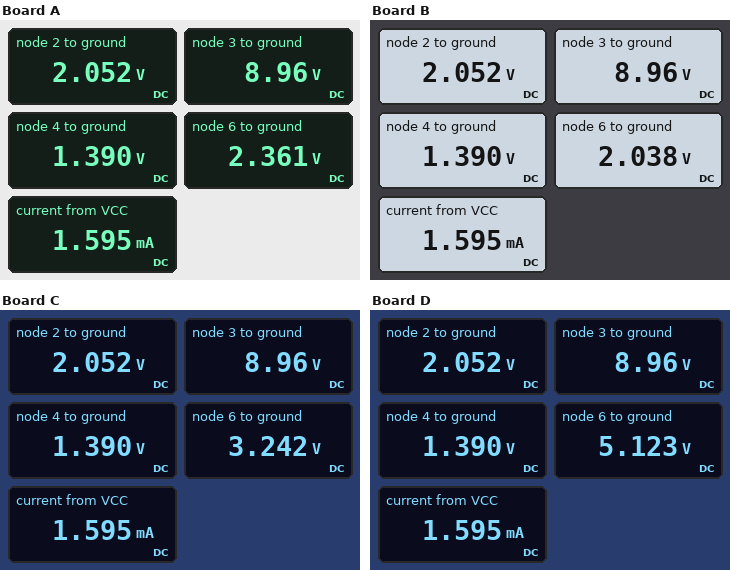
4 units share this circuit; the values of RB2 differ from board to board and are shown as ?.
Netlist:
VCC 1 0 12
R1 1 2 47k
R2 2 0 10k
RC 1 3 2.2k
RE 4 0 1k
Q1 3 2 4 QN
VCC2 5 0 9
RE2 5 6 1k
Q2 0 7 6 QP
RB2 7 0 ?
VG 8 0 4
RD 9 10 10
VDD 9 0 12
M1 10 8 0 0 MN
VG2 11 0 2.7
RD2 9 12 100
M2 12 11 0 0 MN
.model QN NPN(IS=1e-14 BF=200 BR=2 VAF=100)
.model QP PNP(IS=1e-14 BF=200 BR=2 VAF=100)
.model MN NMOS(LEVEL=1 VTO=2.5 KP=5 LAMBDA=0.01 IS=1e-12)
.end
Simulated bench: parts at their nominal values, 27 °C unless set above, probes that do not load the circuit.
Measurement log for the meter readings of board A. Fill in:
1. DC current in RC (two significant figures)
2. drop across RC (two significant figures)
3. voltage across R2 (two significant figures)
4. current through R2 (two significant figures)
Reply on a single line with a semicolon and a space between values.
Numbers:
1.4 mA; 3.0 V; 2.1 V; 210 µA
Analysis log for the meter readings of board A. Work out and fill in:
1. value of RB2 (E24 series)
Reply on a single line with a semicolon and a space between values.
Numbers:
51 kΩ
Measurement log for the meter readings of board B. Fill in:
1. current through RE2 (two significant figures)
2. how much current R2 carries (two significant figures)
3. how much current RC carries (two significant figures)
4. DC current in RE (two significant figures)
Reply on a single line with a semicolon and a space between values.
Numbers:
7.0 mA; 210 µA; 1.4 mA; 1.4 mA
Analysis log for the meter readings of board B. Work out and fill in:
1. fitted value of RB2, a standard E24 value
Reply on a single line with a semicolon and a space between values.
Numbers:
39 kΩ
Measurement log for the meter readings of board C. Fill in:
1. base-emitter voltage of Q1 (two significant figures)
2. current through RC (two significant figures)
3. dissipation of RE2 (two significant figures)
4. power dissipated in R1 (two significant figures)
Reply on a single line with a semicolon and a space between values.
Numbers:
660 mV; 1.4 mA; 33 mW; 2.1 mW
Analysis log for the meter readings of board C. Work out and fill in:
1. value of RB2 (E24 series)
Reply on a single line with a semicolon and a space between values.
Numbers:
91 kΩ
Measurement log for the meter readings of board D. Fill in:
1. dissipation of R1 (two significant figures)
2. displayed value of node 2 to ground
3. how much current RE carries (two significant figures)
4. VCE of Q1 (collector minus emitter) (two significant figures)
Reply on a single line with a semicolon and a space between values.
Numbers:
2.1 mW; 2.052 V; 1.4 mA; 7.6 V
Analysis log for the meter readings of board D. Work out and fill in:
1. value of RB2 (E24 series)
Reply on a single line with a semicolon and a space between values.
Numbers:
240 kΩ
